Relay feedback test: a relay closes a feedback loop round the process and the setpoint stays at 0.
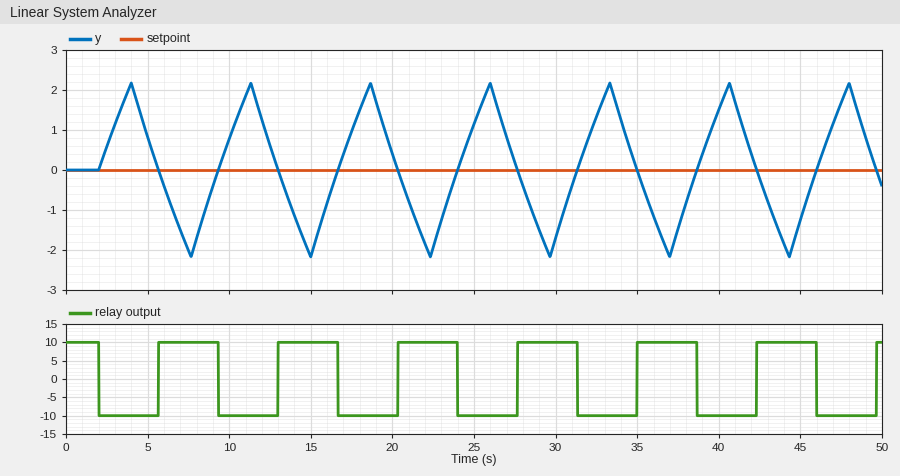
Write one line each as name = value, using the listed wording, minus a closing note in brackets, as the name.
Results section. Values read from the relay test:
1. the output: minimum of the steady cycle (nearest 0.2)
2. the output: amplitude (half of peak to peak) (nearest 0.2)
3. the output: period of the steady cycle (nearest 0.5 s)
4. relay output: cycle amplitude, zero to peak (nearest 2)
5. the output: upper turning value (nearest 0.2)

the output: minimum of the steady cycle = -2.2
the output: amplitude (half of peak to peak) = 2.2
the output: period of the steady cycle = 7.5 s
relay output: cycle amplitude, zero to peak = 10
the output: upper turning value = 2.2
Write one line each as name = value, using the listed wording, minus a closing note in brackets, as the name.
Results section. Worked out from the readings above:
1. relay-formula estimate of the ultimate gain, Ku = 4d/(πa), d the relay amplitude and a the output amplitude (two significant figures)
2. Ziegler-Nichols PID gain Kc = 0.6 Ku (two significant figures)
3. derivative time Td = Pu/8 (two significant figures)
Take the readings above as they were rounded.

relay-formula estimate of the ultimate gain, Ku = 4d/(πa), d the relay amplitude and a the output amplitude = 5.8
Ziegler-Nichols PID gain Kc = 0.6 Ku = 3.5
derivative time Td = Pu/8 = 0.94 s
